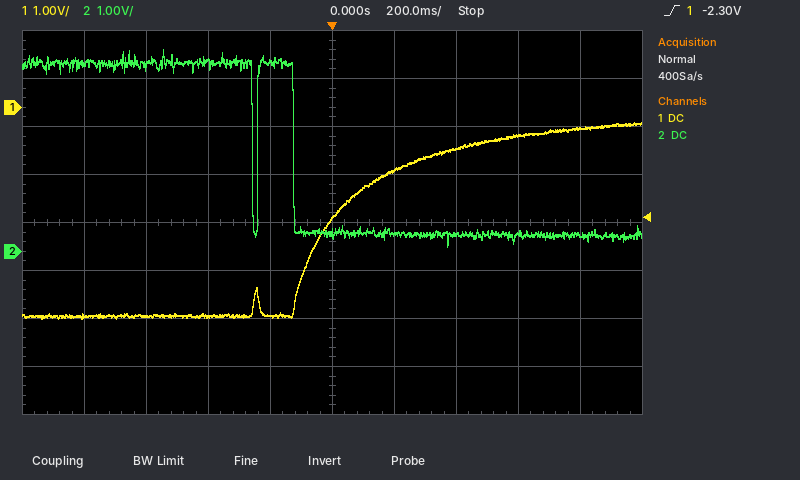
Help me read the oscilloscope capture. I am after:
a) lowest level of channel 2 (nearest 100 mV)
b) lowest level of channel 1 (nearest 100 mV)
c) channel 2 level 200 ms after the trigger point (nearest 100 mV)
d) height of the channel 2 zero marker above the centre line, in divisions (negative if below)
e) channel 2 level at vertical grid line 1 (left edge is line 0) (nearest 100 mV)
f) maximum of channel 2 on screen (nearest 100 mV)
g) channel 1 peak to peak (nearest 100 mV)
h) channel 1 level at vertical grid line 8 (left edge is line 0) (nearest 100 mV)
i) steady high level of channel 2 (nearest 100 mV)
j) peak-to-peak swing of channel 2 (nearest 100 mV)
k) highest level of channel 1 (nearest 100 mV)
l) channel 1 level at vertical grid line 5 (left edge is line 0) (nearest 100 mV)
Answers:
100 mV
-4.4 V
400 mV
-0.6 div
3.9 V
4.2 V
4.1 V
-600 mV
3.9 V
4.1 V
-300 mV
-2.3 V
